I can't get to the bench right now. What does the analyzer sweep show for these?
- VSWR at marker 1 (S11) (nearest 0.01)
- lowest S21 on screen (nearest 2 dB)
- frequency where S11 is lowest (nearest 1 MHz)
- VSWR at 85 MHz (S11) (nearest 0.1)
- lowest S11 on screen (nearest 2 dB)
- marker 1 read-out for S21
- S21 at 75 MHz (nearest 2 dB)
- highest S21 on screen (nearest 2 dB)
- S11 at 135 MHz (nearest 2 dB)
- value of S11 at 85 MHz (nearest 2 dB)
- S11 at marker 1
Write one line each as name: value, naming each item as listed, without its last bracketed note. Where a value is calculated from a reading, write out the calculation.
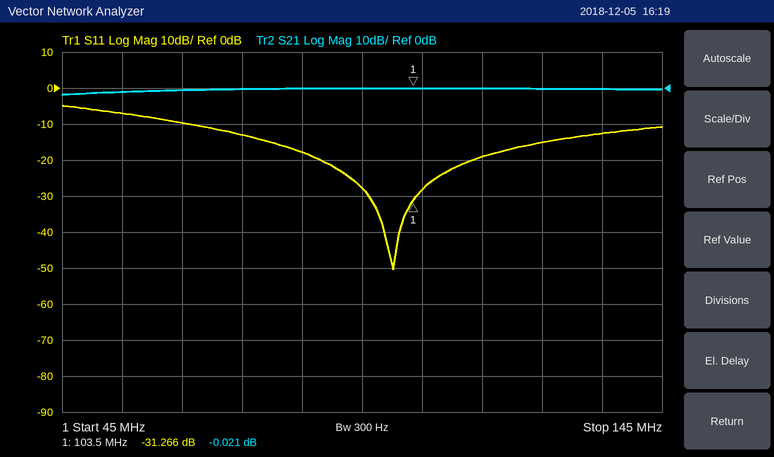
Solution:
VSWR at marker 1 (S11): (1 + 0.0273)/(1 − 0.0273) ≈ 1.06
lowest S21 on screen: -2 dB
frequency where S11 is lowest: 100 MHz
VSWR at 85 MHz (S11): |Γ| = 10^(-18/20) = 0.1259; VSWR = (1 + 0.1259)/(1 − 0.1259) ≈ 1.3
lowest S11 on screen: -50 dB
marker 1 read-out for S21: -0.021 dB
S21 at 75 MHz: 0 dB
highest S21 on screen: 0 dB
S11 at 135 MHz: -12 dB
value of S11 at 85 MHz: -18 dB
S11 at marker 1: -31.266 dB
